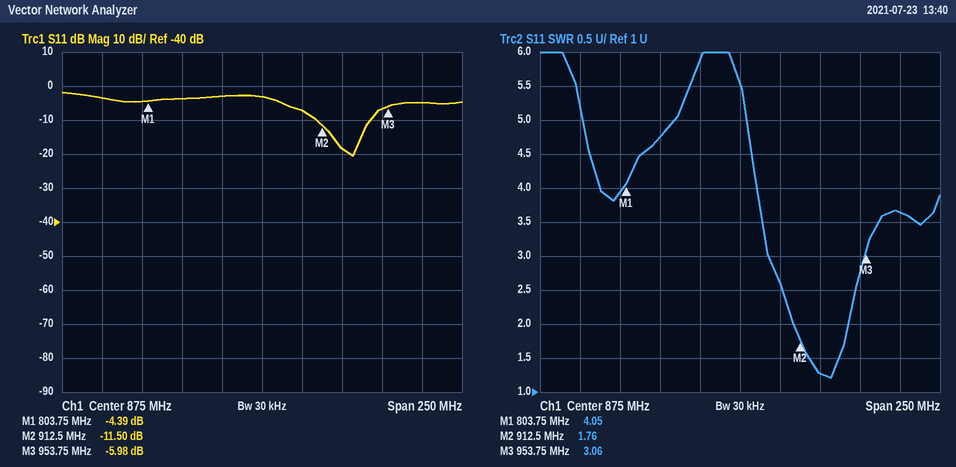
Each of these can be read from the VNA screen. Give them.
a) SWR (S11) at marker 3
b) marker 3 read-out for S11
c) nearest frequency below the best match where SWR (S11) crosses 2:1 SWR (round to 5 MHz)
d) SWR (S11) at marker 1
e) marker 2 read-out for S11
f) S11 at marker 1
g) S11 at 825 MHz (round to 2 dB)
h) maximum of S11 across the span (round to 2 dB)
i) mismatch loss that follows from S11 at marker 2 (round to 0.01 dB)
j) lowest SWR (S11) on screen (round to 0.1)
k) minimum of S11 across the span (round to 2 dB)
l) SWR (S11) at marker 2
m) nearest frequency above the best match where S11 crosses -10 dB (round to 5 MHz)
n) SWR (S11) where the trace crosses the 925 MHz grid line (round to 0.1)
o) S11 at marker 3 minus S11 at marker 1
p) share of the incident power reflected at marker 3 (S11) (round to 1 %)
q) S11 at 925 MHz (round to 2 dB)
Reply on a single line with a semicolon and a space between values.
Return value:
3.06; -5.98 dB; 910 MHz; 4.05; -11.50 dB; -4.39 dB; -4 dB; -2 dB; 0.32 dB; 1.2; -20 dB; 1.76; 945 MHz; 1.3; -1.59 dB; 25 %; -18 dB
